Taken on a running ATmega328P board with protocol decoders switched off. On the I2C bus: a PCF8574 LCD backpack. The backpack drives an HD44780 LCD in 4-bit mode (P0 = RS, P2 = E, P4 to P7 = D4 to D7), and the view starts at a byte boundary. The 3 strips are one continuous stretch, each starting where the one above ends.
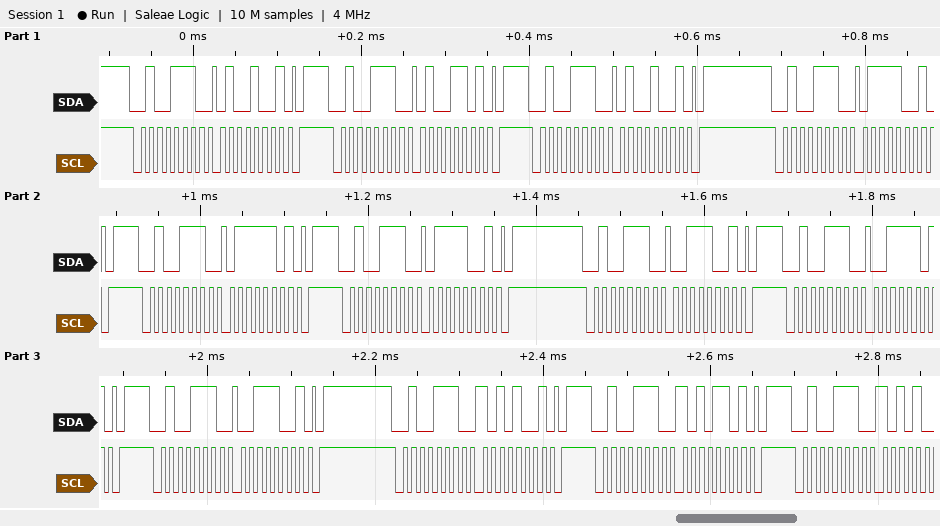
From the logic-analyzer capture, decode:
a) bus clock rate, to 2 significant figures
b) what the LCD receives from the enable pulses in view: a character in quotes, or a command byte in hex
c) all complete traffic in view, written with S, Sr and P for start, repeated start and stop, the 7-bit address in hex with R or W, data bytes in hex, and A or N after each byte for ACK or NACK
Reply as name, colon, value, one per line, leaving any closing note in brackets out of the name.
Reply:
bus clock rate, to 2 significant figures: 100 kHz
what the LCD receives from the enable pulses in view: a character in quotes, or a command byte in hex: 'G'
all complete traffic in view, written with S, Sr and P for start, repeated start and stop, the 7-bit address in hex with R or W, data bytes in hex, and A or N after each byte for ACK or NACK: S 27W A 49 A P S 27W A 4D A P S 27W A 49 A P S 27W A 79 A P S 27W A 7D A P S 27W A 79 A P S 27W A 39 A P S 27W A 3D A P S 27W A 39 A P S 27W A A9 A P S 27W A AD A P S 27W A
